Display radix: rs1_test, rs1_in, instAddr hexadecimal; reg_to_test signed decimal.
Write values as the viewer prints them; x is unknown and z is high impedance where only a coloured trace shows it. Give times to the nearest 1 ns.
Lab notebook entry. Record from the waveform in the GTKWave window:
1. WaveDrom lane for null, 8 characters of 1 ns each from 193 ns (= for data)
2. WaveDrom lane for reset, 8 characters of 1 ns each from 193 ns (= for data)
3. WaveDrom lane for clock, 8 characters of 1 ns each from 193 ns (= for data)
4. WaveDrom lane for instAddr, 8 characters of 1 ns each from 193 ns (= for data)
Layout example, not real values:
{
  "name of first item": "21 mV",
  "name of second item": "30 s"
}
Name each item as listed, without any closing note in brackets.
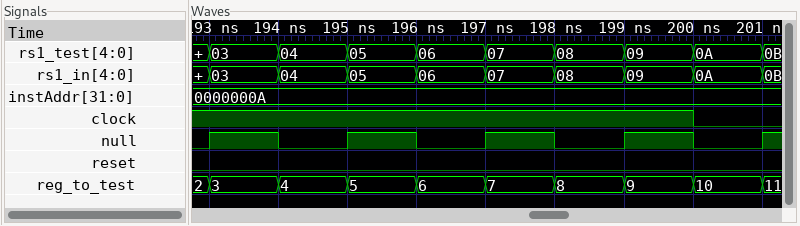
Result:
{
  "WaveDrom lane for null, 8 characters of 1 ns each from 193 ns": "{name: 'null', wave: '10101010'}",
  "WaveDrom lane for reset, 8 characters of 1 ns each from 193 ns": "{name: 'reset', wave: '0.......'}",
  "WaveDrom lane for clock, 8 characters of 1 ns each from 193 ns": "{name: 'clock', wave: '1......0'}",
  "WaveDrom lane for instAddr, 8 characters of 1 ns each from 193 ns": "{name: 'instAddr', wave: '=.......', data: '0000000A'}"
}
